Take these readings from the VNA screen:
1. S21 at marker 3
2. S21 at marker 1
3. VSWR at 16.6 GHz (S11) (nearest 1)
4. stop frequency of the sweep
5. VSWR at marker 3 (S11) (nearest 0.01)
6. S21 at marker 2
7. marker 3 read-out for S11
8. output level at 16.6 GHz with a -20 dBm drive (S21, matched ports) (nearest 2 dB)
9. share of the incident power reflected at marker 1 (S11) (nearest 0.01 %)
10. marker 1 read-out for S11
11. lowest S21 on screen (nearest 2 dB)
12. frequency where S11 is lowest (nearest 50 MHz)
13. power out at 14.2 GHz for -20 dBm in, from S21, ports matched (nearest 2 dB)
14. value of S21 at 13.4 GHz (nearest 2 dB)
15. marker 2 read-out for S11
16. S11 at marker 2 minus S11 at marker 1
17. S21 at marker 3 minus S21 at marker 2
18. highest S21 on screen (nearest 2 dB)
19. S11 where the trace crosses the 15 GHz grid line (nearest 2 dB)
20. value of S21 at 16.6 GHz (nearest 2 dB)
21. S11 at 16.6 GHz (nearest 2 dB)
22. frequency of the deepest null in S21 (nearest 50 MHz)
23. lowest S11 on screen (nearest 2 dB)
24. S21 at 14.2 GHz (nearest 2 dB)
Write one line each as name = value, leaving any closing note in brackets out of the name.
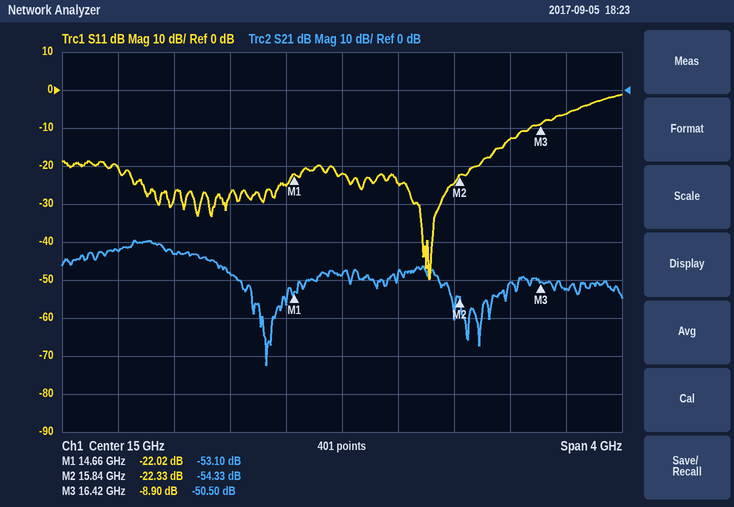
S21 at marker 3 = -50.50 dB
S21 at marker 1 = -53.10 dB
VSWR at 16.6 GHz (S11) = 3
stop frequency of the sweep = 17 GHz
VSWR at marker 3 (S11) = 2.12
S21 at marker 2 = -54.33 dB
marker 3 read-out for S11 = -8.90 dB
output level at 16.6 GHz with a -20 dBm drive (S21, matched ports) = -72 dBm
share of the incident power reflected at marker 1 (S11) = 0.63 %
marker 1 read-out for S11 = -22.02 dB
lowest S21 on screen = -72 dB
frequency where S11 is lowest = 15.60 GHz
power out at 14.2 GHz for -20 dBm in, from S21, ports matched = -68 dBm
value of S21 at 13.4 GHz = -42 dB
marker 2 read-out for S11 = -22.33 dB
S11 at marker 2 minus S11 at marker 1 = -0.31 dB
S21 at marker 3 minus S21 at marker 2 = 3.83 dB
highest S21 on screen = -40 dB
S11 where the trace crosses the 15 GHz grid line = -22 dB
value of S21 at 16.6 GHz = -52 dB
S11 at 16.6 GHz = -6 dB
frequency of the deepest null in S21 = 14.45 GHz
lowest S11 on screen = -50 dB
S21 at 14.2 GHz = -48 dB
